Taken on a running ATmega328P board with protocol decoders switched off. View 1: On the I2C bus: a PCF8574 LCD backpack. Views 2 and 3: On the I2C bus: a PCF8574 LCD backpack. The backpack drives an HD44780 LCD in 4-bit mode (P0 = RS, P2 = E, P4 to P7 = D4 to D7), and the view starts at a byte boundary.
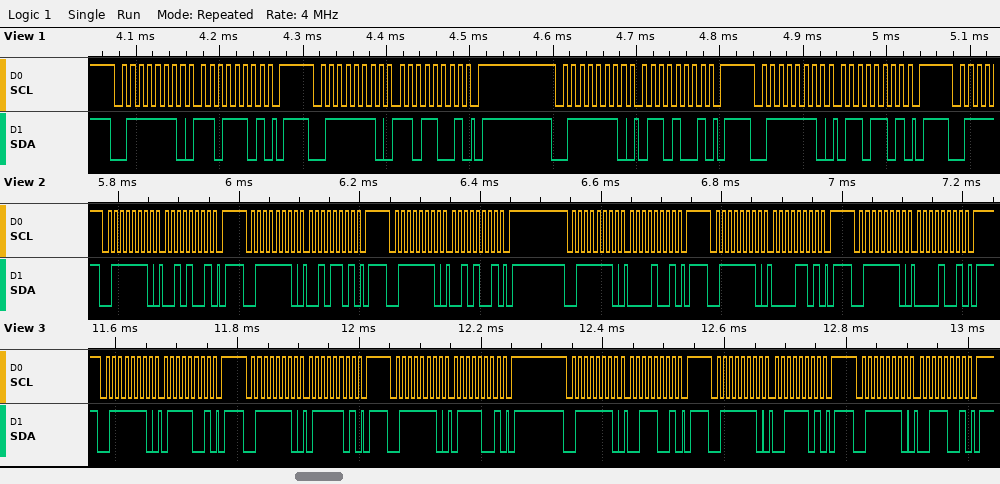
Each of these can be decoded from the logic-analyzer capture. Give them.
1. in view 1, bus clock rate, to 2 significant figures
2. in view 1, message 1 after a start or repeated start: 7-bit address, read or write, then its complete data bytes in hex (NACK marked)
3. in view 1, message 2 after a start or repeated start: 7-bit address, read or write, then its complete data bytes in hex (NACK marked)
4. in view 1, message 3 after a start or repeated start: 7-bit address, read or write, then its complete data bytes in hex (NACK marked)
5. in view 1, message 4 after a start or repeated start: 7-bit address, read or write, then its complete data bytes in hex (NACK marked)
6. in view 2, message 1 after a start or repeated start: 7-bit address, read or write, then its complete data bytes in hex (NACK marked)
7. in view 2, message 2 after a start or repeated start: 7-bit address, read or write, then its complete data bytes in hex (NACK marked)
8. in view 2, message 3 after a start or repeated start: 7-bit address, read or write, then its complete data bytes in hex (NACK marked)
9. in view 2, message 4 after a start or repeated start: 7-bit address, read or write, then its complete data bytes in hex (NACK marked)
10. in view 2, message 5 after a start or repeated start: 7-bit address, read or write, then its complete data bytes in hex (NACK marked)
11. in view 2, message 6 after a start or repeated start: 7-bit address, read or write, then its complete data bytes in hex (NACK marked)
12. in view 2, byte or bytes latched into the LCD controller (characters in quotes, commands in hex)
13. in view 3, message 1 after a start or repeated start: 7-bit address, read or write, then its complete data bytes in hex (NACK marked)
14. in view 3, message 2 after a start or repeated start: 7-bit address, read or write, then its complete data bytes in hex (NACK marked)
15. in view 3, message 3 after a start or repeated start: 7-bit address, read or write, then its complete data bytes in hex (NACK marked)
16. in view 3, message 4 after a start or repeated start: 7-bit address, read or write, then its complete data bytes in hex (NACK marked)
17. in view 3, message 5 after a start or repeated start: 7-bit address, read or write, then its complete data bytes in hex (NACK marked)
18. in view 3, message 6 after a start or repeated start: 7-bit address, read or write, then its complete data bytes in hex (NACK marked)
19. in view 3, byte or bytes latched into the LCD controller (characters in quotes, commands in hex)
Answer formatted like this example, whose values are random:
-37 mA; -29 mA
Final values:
100 kHz; 0x3F write: DD; 0x3F write: D9; 0x3F write: 69; 0x3F write: 6D; 0x3F write: 29; 0x3F write: 2D; 0x3F write: 29; 0x3F write: 09; 0x3F write: 0D; 0x3F write: 09; ' '; 0x3F write: 79; 0x3F write: 7D; 0x3F write: 79; 0x3F write: 39; 0x3F write: 3D; 0x3F write: 39; 's'
